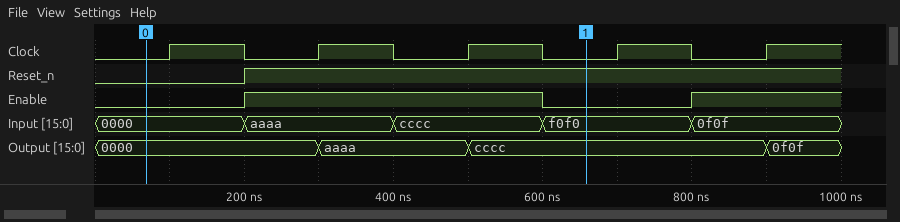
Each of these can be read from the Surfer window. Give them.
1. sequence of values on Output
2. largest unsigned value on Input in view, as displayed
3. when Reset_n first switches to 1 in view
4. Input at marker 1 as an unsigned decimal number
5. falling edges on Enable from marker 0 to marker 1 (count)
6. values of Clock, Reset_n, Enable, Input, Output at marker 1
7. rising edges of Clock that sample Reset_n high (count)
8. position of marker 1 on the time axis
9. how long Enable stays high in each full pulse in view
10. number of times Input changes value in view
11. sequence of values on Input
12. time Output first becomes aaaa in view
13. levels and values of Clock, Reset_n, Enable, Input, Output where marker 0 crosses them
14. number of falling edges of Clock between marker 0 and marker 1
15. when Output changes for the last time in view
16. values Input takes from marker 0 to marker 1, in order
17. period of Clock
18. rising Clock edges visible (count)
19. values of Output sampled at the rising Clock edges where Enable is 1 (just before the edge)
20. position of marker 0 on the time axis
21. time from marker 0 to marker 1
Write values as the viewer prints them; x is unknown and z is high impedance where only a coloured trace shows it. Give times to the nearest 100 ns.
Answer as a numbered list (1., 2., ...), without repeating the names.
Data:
1. 0000, aaaa, cccc, 0f0f
2. f0f0
3. 200 ns
4. 61680
5. 1
6. Clock=0, Reset_n=1, Enable=0, Input=f0f0, Output=cccc
7. 4
8. 700 ns
9. 400 ns
10. 4
11. 0000, aaaa, cccc, f0f0, 0f0f
12. 300 ns
13. Clock=0, Reset_n=0, Enable=0, Input=0000, Output=0000
14. 3
15. 900 ns
16. 0000, aaaa, cccc, f0f0
17. 200 ns
18. 5
19. 0000, aaaa, cccc
20. 100 ns
21. 600 ns
